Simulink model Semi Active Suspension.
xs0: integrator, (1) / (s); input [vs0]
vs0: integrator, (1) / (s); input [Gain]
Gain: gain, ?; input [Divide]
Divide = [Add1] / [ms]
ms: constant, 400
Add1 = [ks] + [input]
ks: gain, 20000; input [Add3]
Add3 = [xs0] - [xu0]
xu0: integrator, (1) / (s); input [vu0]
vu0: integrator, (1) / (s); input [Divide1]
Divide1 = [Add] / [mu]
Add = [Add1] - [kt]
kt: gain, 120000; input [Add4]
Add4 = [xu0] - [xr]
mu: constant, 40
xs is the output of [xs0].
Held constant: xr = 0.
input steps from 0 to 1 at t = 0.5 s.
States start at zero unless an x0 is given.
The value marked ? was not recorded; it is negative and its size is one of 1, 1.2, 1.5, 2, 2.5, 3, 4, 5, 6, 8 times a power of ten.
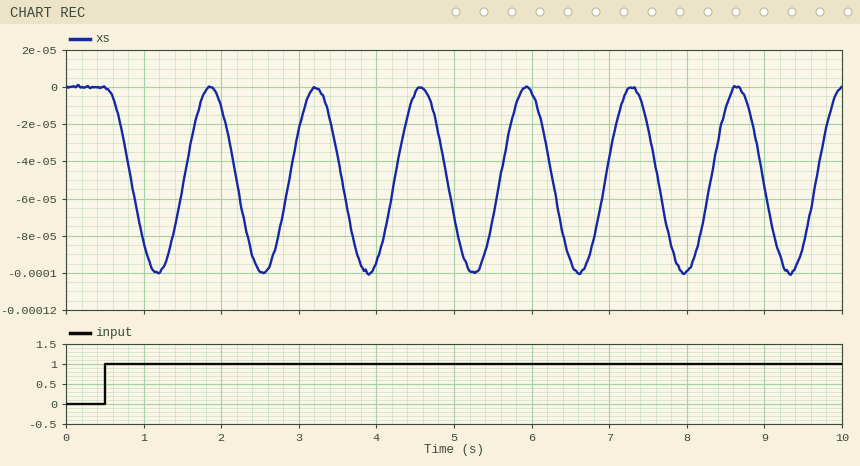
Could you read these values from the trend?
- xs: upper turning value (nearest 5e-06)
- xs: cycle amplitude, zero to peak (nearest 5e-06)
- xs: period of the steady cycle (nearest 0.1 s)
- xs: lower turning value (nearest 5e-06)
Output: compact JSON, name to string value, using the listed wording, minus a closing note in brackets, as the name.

{"xs: upper turning value": "0.000000", "xs: cycle amplitude, zero to peak": "0.000050", "xs: period of the steady cycle": "1.4 s", "xs: lower turning value": "-0.000100"}
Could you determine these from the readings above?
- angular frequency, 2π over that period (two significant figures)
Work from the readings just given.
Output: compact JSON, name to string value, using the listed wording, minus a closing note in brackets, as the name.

{"angular frequency, 2π over that period": "4.5 rad/s"}
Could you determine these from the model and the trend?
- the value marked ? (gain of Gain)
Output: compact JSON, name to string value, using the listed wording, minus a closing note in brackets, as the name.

{"the value marked ?": "-0.5"}
